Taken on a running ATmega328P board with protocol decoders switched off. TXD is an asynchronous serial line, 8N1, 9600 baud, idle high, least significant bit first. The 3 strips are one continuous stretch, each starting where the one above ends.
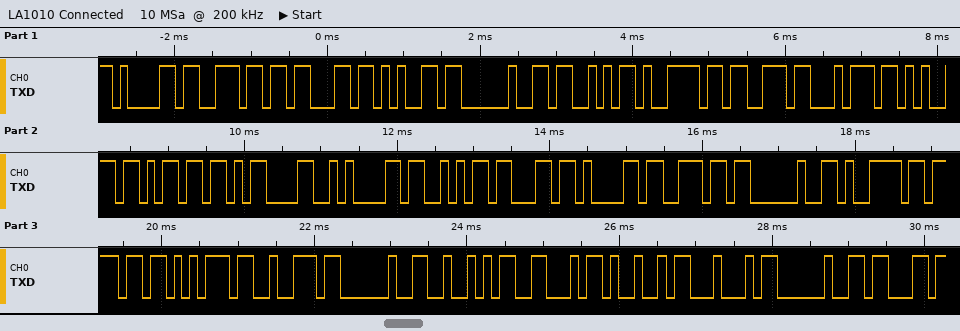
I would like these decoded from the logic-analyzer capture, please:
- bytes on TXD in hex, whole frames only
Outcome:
61 6E 63 65 20 53 79 73 74 65 6D 0D 0A 53 63 61 6E 20 79 6F 75 72 20 52 46 49 44 20 63
